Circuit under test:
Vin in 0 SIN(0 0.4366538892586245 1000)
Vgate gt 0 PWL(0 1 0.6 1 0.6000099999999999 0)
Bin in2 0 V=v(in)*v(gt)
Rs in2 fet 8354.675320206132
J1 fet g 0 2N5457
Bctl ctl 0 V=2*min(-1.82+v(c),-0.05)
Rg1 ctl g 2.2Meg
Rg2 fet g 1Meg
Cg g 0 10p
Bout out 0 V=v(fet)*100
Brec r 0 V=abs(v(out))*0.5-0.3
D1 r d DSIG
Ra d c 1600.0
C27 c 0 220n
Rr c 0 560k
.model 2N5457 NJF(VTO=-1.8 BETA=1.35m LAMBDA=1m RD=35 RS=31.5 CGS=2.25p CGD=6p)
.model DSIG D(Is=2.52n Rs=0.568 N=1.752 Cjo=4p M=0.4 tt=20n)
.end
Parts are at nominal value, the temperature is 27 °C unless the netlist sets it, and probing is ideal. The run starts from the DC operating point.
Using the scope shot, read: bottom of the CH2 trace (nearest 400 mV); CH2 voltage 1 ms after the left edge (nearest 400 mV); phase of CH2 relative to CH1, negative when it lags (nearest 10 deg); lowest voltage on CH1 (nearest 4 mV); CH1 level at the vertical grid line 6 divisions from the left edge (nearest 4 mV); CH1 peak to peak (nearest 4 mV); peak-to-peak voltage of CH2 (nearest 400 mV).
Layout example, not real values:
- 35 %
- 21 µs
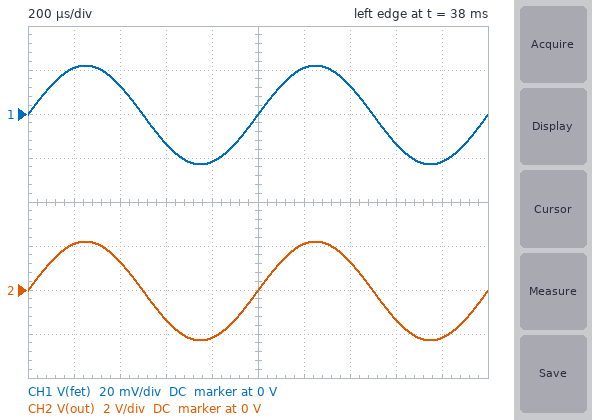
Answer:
- -2.4 V
- 0 V
- 0 deg
- -24 mV
- 20 mV
- 44 mV
- 4.4 V
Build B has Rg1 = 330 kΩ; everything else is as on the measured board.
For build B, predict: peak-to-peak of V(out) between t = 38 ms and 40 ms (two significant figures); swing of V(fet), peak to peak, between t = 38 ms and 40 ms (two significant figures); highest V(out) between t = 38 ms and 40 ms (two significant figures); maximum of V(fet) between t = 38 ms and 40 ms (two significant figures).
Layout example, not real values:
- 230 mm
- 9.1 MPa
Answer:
- 6.8 V
- 68 mV
- 3.4 V
- 34 mV
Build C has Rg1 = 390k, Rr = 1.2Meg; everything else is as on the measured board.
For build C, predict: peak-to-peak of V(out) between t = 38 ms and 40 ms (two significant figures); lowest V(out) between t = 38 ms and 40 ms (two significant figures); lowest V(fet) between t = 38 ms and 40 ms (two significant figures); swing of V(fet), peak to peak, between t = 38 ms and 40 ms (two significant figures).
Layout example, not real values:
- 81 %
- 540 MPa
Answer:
- 6.6 V
- -3.3 V
- -33 mV
- 66 mV
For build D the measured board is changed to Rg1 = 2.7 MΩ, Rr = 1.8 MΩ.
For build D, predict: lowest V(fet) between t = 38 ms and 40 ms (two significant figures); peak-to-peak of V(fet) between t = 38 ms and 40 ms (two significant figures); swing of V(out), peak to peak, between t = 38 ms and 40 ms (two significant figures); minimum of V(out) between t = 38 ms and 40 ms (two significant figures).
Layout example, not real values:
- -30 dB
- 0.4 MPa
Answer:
- -21 mV
- 42 mV
- 4.2 V
- -2.1 V
